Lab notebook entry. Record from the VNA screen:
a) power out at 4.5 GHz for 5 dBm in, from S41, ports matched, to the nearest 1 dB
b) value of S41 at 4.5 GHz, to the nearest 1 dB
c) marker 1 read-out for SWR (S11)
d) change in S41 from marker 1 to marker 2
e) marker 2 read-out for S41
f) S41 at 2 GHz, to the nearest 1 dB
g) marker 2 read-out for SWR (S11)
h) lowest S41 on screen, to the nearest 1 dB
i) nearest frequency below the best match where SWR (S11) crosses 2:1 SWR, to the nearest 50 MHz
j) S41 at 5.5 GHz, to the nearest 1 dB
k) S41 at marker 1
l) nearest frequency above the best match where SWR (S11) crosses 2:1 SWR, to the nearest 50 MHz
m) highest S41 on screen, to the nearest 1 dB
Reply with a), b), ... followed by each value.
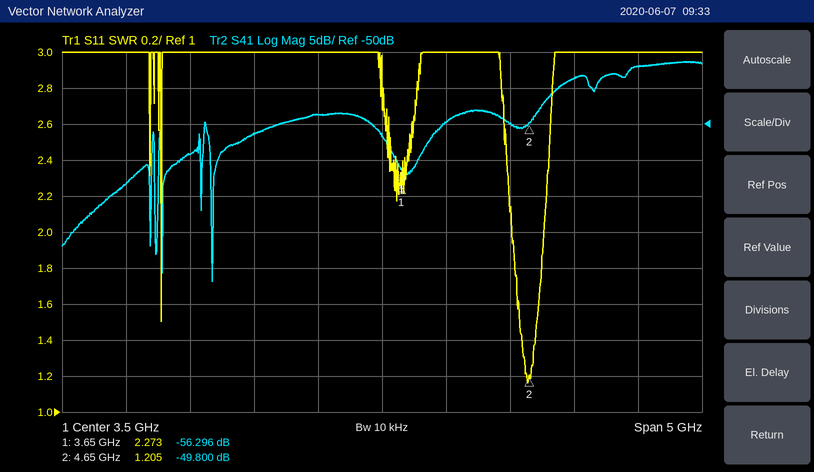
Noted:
a) -45 dBm
b) -50 dB
c) 2.273
d) 6.496 dB
e) -49.800 dB
f) -54 dB
g) 1.205
h) -72 dB
i) 4.50 GHz
j) -42 dB
k) -56.296 dB
l) 4.75 GHz
m) -41 dB
